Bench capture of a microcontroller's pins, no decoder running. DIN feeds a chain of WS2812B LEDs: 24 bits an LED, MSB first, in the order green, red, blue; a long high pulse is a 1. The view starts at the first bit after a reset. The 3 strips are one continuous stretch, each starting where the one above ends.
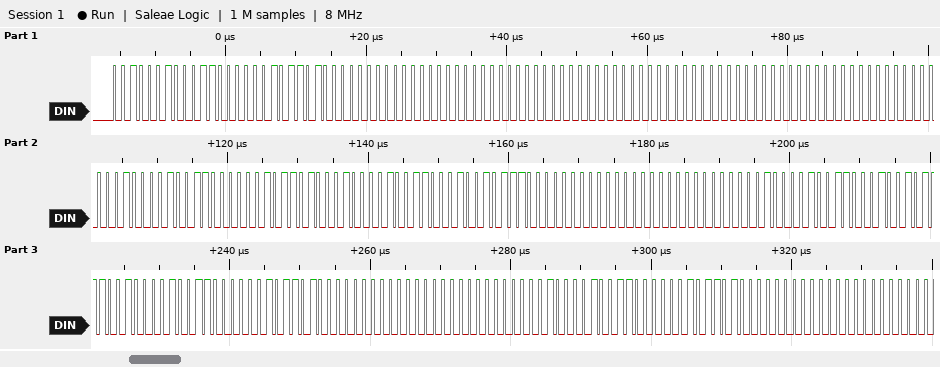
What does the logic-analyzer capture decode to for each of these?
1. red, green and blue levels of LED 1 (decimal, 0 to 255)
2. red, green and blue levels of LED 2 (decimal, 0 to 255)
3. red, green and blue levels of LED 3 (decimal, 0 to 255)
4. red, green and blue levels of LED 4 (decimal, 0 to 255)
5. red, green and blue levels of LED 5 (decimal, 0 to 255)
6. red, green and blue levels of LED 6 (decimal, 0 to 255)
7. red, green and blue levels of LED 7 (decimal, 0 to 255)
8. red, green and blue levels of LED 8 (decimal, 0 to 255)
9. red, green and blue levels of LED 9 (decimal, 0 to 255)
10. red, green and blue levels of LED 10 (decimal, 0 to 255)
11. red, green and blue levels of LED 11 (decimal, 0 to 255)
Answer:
48, 34, 45
0, 0, 0
0, 0, 0
0, 0, 0
96, 66, 90
49, 33, 46
0, 0, 0
49, 33, 46
96, 66, 90
0, 0, 0
96, 66, 90
